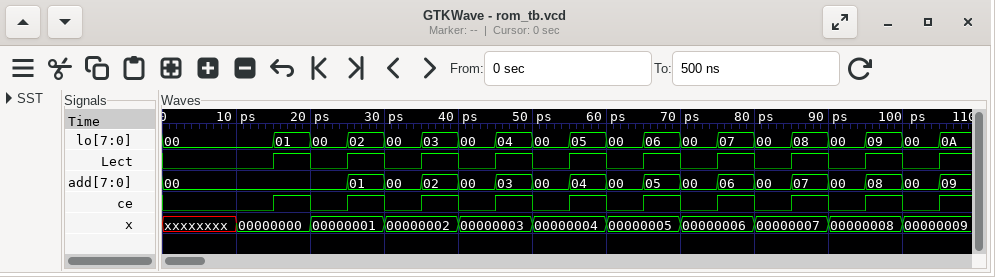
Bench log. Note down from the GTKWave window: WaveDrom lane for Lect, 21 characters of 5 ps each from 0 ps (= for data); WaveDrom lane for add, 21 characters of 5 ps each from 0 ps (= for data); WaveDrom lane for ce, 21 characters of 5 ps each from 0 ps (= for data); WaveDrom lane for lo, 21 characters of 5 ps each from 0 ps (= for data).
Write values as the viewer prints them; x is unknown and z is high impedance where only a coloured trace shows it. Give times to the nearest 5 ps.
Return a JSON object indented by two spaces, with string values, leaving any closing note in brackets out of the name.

{
  "WaveDrom lane for Lect, 21 characters of 5 ps each from 0 ps": "{name: 'Lect', wave: '0..101010101010101010'}",
  "WaveDrom lane for add, 21 characters of 5 ps each from 0 ps": "{name: 'add', wave: '=....================', data: '00 01 00 02 00 03 00 04 00 05 00 06 00 07 00 08 00'}",
  "WaveDrom lane for ce, 21 characters of 5 ps each from 0 ps": "{name: 'ce', wave: '0..101010101010101010'}",
  "WaveDrom lane for lo, 21 characters of 5 ps each from 0 ps": "{name: 'lo', wave: '=..==================', data: '00 01 00 02 00 03 00 04 00 05 00 06 00 07 00 08 00 09 00'}"
}
